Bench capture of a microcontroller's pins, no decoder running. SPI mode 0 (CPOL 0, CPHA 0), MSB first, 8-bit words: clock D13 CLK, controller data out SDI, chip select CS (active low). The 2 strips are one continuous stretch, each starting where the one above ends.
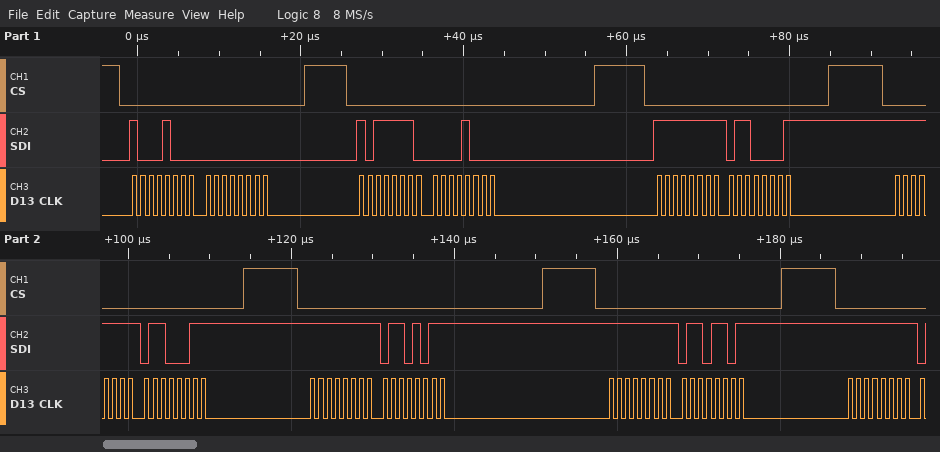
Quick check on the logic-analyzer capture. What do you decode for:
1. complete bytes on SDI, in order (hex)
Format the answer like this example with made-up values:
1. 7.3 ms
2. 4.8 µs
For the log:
1. 88 00 BE 08 FF 61 FF 63 FF 6B FF 6D FF
